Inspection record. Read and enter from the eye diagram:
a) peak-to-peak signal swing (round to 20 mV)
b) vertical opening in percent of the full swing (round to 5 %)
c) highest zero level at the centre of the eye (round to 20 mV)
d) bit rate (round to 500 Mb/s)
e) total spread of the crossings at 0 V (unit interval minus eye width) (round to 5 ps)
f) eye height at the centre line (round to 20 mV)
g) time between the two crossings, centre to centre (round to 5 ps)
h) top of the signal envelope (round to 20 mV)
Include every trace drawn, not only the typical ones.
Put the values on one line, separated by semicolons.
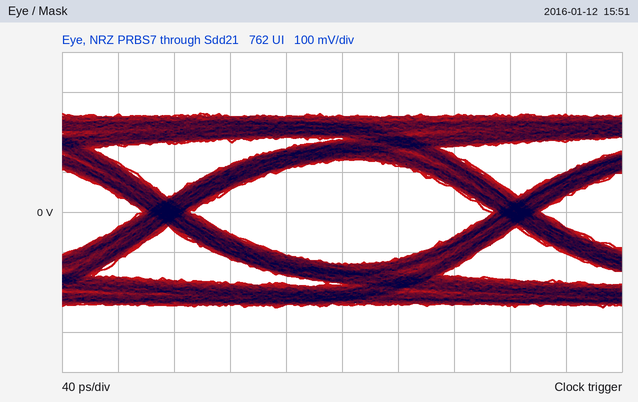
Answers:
480 mV; 55 %; -140 mV; 4.0 Gb/s; 35 ps; 260 mV; 250 ps; 240 mV
